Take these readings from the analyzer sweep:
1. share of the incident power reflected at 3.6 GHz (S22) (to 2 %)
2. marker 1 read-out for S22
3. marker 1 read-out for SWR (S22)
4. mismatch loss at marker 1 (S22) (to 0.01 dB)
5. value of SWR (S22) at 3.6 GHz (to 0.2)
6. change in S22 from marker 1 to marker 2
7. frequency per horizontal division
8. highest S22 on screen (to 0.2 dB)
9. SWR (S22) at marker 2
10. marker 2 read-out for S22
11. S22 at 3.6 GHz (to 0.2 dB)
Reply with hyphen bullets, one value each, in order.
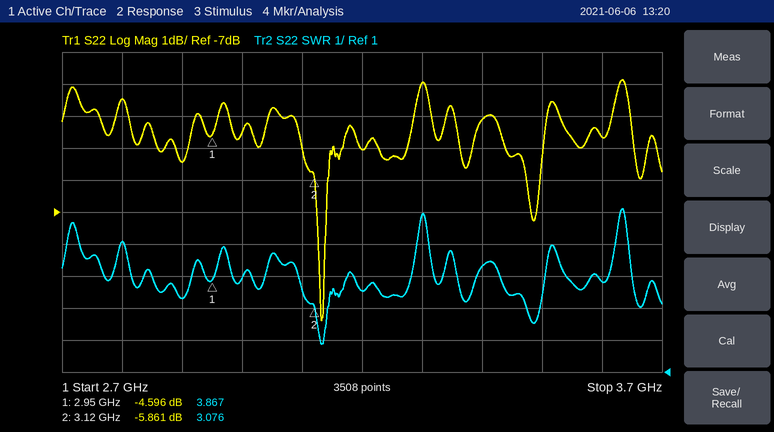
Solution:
- 34 %
- -4.596 dB
- 3.867
- 1.85 dB
- 3.8
- -1.265 dB
- 100 MHz
- -2.8 dB
- 3.076
- -5.861 dB
- -4.6 dB
